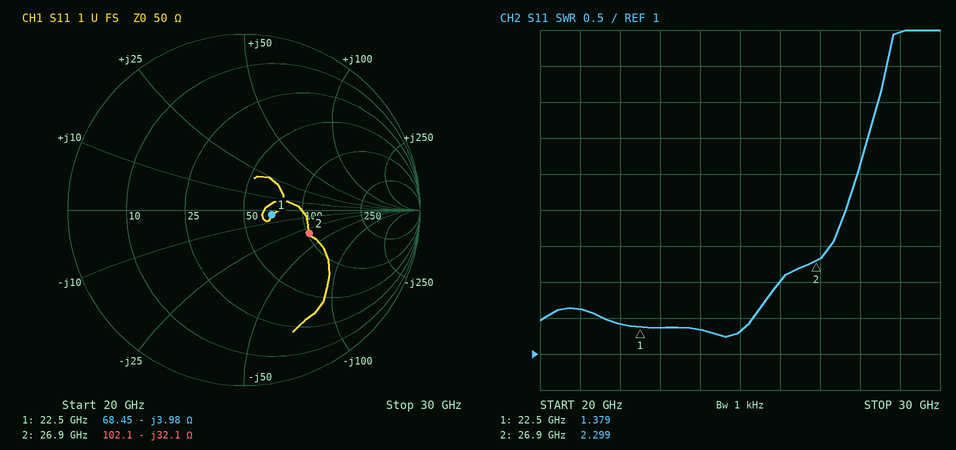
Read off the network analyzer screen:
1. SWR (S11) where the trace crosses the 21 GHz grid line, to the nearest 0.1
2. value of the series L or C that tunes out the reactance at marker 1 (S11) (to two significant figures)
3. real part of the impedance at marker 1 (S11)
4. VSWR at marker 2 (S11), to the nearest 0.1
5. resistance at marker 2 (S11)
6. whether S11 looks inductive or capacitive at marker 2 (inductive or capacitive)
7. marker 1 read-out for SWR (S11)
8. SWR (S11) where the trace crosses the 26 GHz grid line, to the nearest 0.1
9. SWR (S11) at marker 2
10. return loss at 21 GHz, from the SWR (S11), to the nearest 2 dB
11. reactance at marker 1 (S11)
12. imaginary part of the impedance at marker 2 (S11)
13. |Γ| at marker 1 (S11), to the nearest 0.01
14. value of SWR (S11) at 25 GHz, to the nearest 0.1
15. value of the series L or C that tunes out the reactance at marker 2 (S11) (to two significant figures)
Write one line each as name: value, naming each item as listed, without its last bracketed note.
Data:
SWR (S11) where the trace crosses the 21 GHz grid line, to the nearest 0.1: 1.6
value of the series L or C that tunes out the reactance at marker 1 (S11): 28 pH
real part of the impedance at marker 1: 68.45 Ω
VSWR at marker 2 (S11), to the nearest 0.1: 2.3
resistance at marker 2: 102.1 Ω
whether S11 looks inductive or capacitive at marker 2: capacitive
marker 1 read-out for SWR: 1.379
SWR (S11) where the trace crosses the 26 GHz grid line, to the nearest 0.1: 2.0
SWR (S11) at marker 2: 2.299
return loss at 21 GHz, from the SWR (S11), to the nearest 2 dB: 12 dB
reactance at marker 1: -3.98 Ω
imaginary part of the impedance at marker 2: -32.1 Ω
|Γ| at marker 1 (S11), to the nearest 0.01: 0.16
value of SWR (S11) at 25 GHz, to the nearest 0.1: 1.3
value of the series L or C that tunes out the reactance at marker 2 (S11): 190 pH
